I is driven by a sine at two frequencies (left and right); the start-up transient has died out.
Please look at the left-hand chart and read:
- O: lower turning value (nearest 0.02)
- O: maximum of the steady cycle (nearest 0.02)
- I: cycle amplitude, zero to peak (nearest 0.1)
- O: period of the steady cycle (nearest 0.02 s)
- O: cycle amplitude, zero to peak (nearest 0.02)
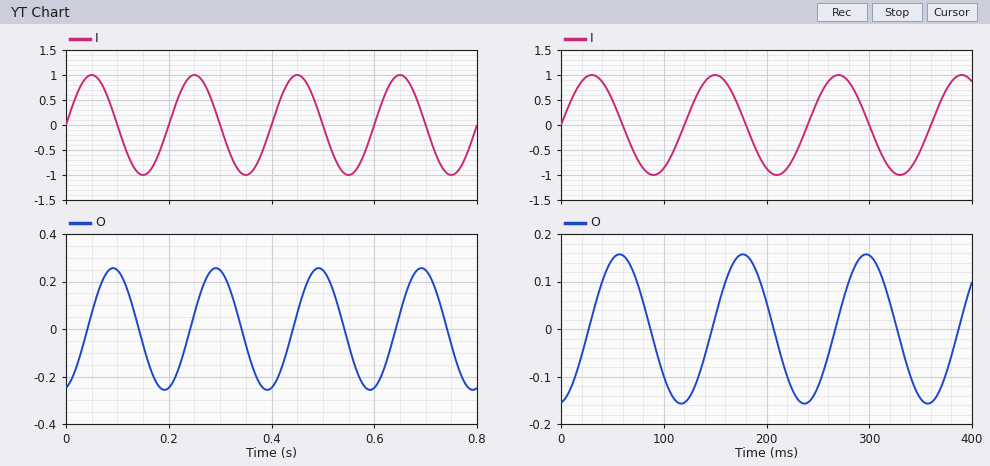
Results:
-0.26
0.26
1.0
0.20 s
0.26
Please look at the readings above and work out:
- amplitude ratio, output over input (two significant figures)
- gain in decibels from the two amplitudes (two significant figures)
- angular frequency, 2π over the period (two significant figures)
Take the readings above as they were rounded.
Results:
0.26
-12 dB
31 rad/s
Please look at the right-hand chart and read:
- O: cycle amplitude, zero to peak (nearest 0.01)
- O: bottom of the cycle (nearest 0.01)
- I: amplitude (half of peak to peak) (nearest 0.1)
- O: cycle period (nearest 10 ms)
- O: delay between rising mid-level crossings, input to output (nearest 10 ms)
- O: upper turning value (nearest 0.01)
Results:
0.16
-0.16
1.0
120 ms
30 ms
0.16
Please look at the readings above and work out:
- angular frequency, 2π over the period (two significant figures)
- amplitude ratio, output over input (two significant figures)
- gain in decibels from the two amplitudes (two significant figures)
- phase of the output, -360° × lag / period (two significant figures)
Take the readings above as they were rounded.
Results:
0.052 rad/ms
0.16
-16 dB
-90°
